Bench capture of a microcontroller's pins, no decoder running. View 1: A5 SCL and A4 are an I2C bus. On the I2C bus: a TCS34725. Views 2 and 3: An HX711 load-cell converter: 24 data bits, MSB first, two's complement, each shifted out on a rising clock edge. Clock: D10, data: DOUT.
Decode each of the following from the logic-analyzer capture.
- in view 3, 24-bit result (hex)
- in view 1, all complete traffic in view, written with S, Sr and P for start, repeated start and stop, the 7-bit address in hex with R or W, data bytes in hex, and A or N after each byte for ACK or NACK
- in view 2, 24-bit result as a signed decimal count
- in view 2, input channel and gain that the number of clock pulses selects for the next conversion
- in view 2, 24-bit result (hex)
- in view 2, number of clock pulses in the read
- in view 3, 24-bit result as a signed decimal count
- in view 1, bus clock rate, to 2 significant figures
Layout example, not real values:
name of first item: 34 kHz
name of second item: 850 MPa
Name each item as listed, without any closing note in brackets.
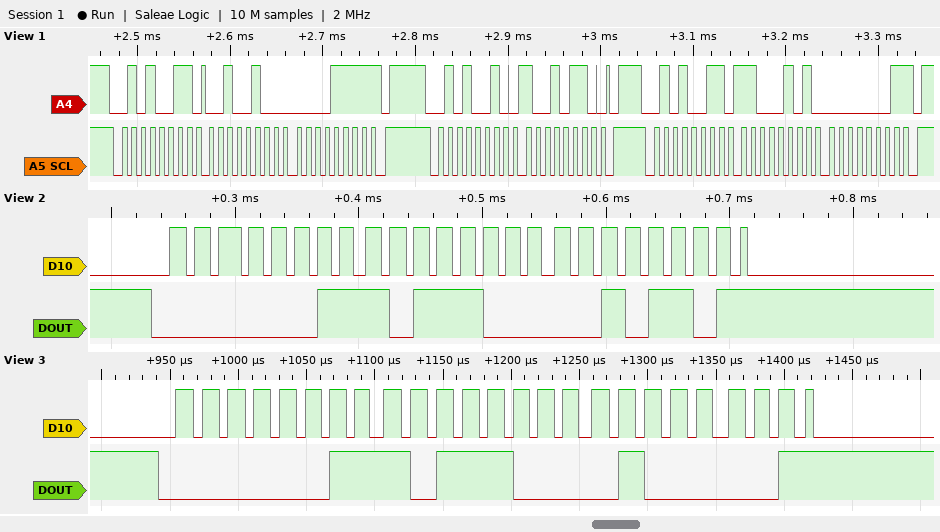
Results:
in view 3, 24-bit result: 0x03B841
in view 1, all complete traffic in view, written with S, Sr and P for start, repeated start and stop, the 7-bit address in hex with R or W, data bytes in hex, and A or N after each byte for ACK or NACK: S 29R A 24 A 0F N P S 29W A 96 A P S 29R A C5 A 01 N P
in view 2, 24-bit result as a signed decimal count: 243757
in view 2, input channel and gain that the number of clock pulses selects for the next conversion: channel A, gain 128
in view 2, 24-bit result: 0x03B82D
in view 2, number of clock pulses in the read: 25
in view 3, 24-bit result as a signed decimal count: 243777
in view 1, bus clock rate, to 2 significant figures: 100 kHz
